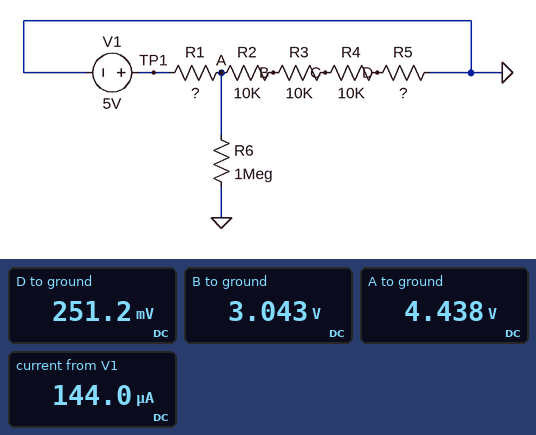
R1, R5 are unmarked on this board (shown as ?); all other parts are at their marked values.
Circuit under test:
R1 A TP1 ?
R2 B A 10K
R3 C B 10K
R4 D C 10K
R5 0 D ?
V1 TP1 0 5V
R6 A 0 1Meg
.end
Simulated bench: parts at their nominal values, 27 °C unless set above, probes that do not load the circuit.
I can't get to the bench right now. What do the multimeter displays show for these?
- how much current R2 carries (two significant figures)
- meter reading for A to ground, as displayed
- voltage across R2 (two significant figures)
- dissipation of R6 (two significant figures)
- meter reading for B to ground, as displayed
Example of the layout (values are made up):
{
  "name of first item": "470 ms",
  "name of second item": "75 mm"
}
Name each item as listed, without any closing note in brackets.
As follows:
{
  "how much current R2 carries": "140 µA",
  "meter reading for A to ground, as displayed": "4.438 V",
  "voltage across R2": "1.4 V",
  "dissipation of R6": "20 µW",
  "meter reading for B to ground, as displayed": "3.043 V"
}
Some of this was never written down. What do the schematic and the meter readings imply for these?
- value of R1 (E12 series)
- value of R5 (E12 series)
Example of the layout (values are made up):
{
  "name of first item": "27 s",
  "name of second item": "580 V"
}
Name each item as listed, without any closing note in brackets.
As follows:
{
  "value of R1": "3.9 kΩ",
  "value of R5": "1.8 kΩ"
}
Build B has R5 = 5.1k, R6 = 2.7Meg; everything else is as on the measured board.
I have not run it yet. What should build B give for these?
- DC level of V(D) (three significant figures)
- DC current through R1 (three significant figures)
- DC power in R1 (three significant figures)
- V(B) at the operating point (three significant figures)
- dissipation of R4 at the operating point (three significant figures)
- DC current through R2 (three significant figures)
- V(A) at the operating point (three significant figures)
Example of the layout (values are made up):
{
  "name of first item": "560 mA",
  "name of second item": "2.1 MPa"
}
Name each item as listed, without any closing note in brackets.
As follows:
{
  "DC level of V(D)": "653 mV",
  "DC current through R1": "130 µA",
  "DC power in R1": "65.6 µW",
  "V(B) at the operating point": "3.21 V",
  "dissipation of R4 at the operating point": "164 µW",
  "DC current through R2": "128 µA",
  "V(A) at the operating point": "4.49 V"
}
